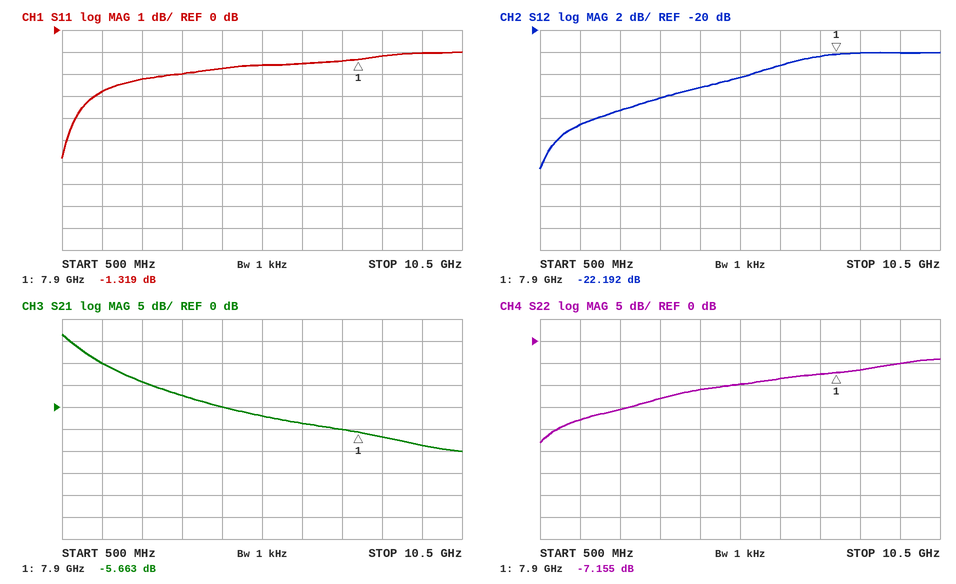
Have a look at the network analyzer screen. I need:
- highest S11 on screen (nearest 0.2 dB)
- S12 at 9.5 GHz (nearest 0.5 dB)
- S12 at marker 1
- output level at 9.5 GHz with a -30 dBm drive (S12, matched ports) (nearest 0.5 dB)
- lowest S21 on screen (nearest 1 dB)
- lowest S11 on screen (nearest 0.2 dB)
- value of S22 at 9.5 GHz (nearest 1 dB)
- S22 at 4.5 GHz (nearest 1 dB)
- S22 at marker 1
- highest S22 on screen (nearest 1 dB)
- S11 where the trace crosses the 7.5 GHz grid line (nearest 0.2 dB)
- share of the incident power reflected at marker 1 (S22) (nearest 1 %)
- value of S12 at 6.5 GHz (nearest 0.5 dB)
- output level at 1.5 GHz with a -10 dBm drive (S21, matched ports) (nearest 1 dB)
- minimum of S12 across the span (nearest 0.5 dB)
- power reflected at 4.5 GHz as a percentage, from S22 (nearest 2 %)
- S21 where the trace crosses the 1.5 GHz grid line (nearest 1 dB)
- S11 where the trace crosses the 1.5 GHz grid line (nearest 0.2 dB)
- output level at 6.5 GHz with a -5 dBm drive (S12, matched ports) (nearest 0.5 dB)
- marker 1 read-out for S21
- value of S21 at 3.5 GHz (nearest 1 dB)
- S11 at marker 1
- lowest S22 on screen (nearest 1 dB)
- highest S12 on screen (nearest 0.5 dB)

-1.0 dB
-22.0 dB
-22.192 dB
-52.0 dBm
-10 dB
-5.8 dB
-5 dB
-11 dB
-7.155 dB
-4 dB
-1.4 dB
19 %
-23.0 dB
0 dBm
-32.5 dB
8 %
10 dB
-2.8 dB
-28.0 dBm
-5.663 dB
3 dB
-1.319 dB
-23 dB
-22.0 dB
